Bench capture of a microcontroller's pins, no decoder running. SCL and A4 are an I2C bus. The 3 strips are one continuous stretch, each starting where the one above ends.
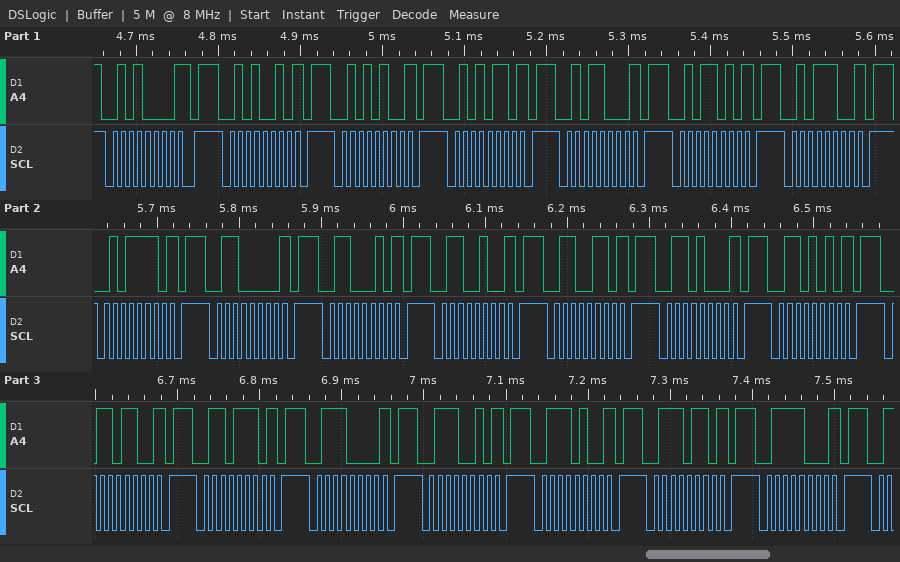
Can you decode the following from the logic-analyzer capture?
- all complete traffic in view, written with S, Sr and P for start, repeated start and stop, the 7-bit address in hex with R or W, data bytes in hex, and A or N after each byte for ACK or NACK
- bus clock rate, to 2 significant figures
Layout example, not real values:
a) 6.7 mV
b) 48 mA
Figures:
a) S 28W N P S 29W N P S 2AW N P S 2BW N P S 2CW N P S 2DW N P S 2EW N P S 2FW N P S 30W N P S 31W N P S 32W N P S 33W N P S 34W N P S 35W N P S 36W N P S 37W N P S 38W N P S 39W N P S 3AW N P S 3BW N P S 3CW N P
b) 100 kHz
